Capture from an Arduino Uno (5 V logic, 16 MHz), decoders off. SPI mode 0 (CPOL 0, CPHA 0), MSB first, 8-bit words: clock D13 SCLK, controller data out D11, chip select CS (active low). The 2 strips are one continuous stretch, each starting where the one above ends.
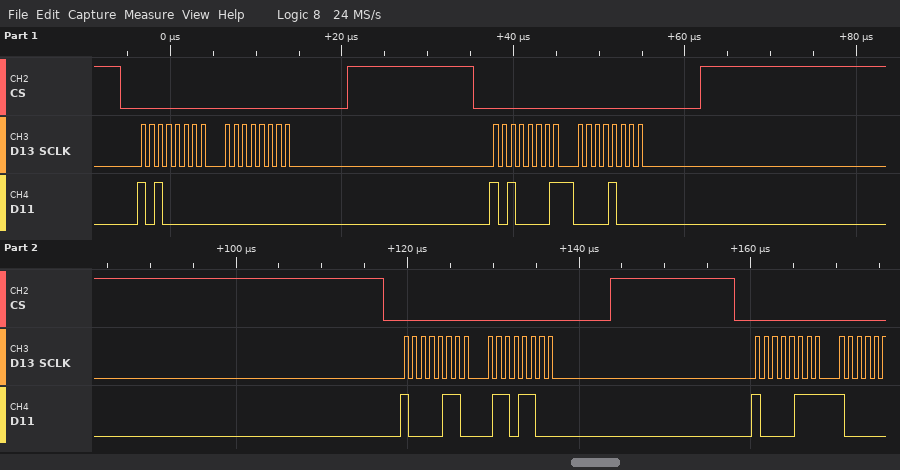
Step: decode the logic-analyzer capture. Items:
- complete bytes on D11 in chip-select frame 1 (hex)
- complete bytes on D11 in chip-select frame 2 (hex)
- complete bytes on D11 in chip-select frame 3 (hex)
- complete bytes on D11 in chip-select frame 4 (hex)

0xA0 0x00
0xA1 0x08
0x86 0x6C
0x87
